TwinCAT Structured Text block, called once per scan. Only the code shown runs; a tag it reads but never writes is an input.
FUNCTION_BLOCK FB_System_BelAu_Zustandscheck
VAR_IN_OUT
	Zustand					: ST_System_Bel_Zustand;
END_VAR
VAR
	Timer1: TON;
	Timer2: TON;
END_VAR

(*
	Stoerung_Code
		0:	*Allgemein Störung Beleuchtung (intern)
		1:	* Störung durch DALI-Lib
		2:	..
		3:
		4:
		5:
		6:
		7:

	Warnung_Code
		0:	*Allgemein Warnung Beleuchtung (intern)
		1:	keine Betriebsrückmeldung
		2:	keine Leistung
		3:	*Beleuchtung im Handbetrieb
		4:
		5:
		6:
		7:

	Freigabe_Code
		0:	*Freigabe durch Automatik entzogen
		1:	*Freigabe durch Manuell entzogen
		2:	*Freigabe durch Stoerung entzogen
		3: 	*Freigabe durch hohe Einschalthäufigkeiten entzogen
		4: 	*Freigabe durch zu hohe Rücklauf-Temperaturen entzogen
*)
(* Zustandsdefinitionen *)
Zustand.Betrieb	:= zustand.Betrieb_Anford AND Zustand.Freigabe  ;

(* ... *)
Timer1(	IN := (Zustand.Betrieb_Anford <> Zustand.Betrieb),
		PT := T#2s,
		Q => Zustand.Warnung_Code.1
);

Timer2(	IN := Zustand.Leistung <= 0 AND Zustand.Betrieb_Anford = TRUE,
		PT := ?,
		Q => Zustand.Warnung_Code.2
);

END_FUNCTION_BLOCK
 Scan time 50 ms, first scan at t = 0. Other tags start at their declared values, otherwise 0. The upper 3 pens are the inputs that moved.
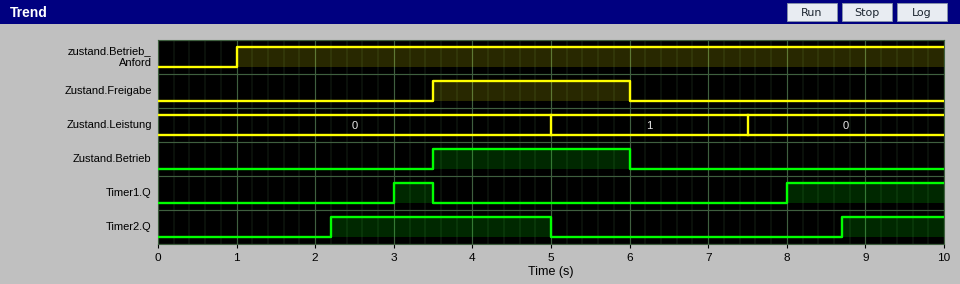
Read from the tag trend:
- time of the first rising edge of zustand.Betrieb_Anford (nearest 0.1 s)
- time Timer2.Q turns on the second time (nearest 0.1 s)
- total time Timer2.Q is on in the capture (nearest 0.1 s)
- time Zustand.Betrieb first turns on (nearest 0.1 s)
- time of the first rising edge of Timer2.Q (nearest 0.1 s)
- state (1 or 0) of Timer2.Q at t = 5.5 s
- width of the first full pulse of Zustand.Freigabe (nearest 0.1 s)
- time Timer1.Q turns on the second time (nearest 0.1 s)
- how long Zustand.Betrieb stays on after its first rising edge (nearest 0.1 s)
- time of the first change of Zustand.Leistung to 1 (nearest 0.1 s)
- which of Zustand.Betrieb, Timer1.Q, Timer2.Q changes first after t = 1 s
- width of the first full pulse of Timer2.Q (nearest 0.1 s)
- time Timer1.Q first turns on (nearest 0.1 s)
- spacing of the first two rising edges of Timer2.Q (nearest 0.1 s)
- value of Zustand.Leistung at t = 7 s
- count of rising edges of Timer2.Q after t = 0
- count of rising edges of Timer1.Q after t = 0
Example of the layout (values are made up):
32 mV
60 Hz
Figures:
1.0 s
8.7 s
4.1 s
3.5 s
2.2 s
0
2.5 s
8.0 s
2.5 s
5.0 s
Timer2.Q
2.8 s
3.0 s
6.5 s
1
2
2
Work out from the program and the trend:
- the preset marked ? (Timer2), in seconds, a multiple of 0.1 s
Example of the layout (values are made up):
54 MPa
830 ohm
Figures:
1.2 s
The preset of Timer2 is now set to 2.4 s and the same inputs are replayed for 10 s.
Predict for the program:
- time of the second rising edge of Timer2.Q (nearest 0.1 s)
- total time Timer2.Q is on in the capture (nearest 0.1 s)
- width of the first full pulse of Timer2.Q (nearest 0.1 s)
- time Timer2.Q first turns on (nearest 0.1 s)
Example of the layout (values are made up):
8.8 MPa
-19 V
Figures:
9.9 s
1.7 s
1.6 s
3.4 s
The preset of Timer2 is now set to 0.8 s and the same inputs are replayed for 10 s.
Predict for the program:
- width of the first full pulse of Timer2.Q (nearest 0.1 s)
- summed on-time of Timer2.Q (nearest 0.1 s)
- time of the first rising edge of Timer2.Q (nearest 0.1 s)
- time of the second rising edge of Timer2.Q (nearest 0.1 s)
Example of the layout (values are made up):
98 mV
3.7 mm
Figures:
3.2 s
4.9 s
1.8 s
8.3 s
